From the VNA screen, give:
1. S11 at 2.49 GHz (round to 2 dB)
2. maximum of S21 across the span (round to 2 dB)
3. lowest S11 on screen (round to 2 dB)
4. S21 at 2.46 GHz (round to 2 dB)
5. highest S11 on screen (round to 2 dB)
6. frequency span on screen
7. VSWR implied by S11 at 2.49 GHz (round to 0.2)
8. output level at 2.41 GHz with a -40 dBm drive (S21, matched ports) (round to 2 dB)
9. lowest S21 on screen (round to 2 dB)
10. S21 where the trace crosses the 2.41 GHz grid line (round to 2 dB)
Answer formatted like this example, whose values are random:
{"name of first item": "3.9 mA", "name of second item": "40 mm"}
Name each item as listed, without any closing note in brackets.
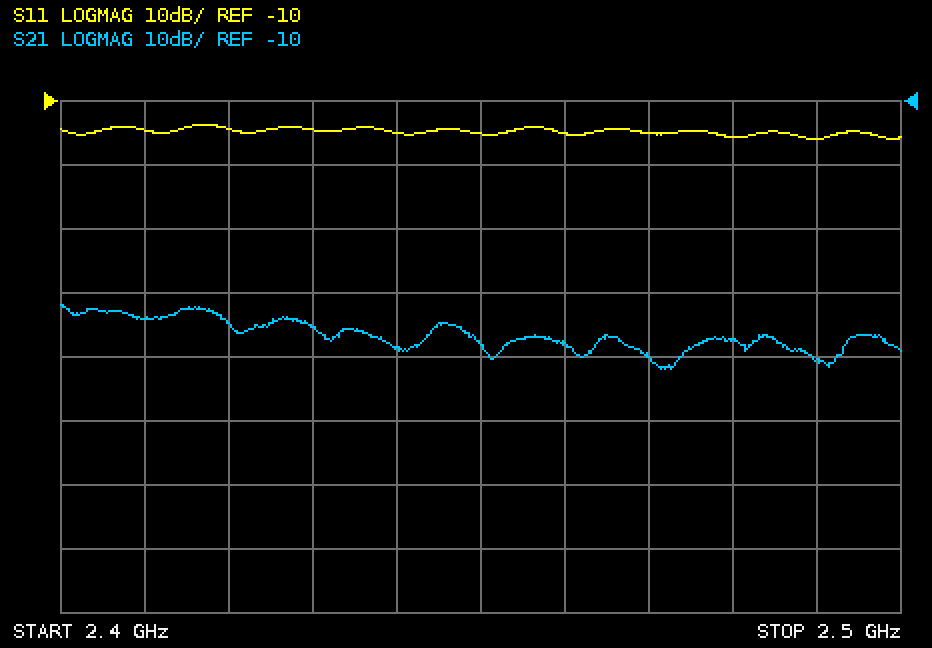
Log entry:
{"S11 at 2.49 GHz": "-16 dB", "maximum of S21 across the span": "-42 dB", "lowest S11 on screen": "-16 dB", "S21 at 2.46 GHz": "-48 dB", "highest S11 on screen": "-14 dB", "frequency span on screen": "100 MHz", "VSWR implied by S11 at 2.49 GHz": "1.4", "output level at 2.41 GHz with a -40 dBm drive (S21, matched ports)": "-84 dBm", "lowest S21 on screen": "-52 dB", "S21 where the trace crosses the 2.41 GHz grid line": "-44 dB"}
